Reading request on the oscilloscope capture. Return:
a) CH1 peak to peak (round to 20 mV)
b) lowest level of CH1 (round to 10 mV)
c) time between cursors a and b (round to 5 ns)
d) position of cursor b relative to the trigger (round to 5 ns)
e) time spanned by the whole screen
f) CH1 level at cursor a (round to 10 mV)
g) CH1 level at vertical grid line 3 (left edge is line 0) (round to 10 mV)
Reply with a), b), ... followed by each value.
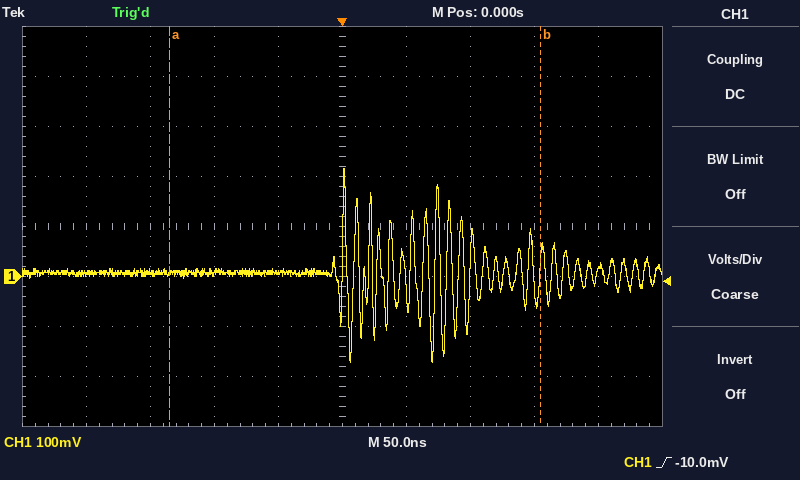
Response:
a) 380 mV
b) -170 mV
c) 290 ns
d) +155 ns
e) 500 ns
f) 10 mV
g) 10 mV
